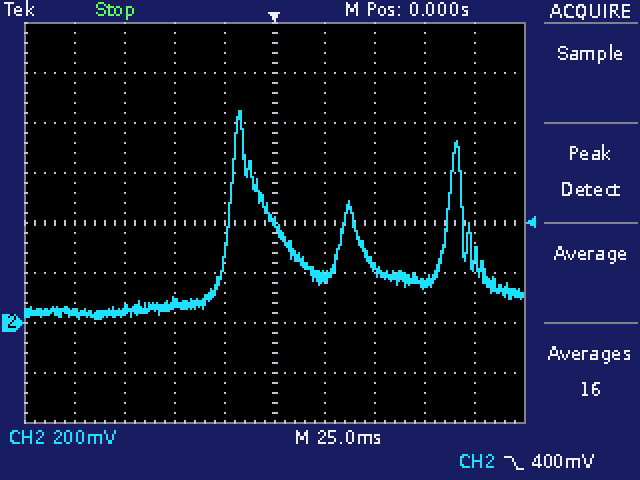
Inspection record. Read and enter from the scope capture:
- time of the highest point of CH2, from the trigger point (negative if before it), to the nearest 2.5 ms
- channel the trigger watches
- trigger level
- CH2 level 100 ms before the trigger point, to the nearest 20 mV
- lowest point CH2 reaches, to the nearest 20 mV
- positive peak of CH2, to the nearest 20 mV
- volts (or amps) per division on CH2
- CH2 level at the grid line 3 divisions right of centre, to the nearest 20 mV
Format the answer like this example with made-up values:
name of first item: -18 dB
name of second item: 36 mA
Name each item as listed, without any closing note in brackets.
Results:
time of the highest point of CH2, from the trigger point (negative if before it), to the nearest 2.5 ms: -17.5 ms
channel the trigger watches: CH2
trigger level: 400 mV
CH2 level 100 ms before the trigger point, to the nearest 20 mV: 40 mV
lowest point CH2 reaches, to the nearest 20 mV: 20 mV
positive peak of CH2, to the nearest 20 mV: 840 mV
volts (or amps) per division on CH2: 200 mV
CH2 level at the grid line 3 divisions right of centre, to the nearest 20 mV: 160 mV
